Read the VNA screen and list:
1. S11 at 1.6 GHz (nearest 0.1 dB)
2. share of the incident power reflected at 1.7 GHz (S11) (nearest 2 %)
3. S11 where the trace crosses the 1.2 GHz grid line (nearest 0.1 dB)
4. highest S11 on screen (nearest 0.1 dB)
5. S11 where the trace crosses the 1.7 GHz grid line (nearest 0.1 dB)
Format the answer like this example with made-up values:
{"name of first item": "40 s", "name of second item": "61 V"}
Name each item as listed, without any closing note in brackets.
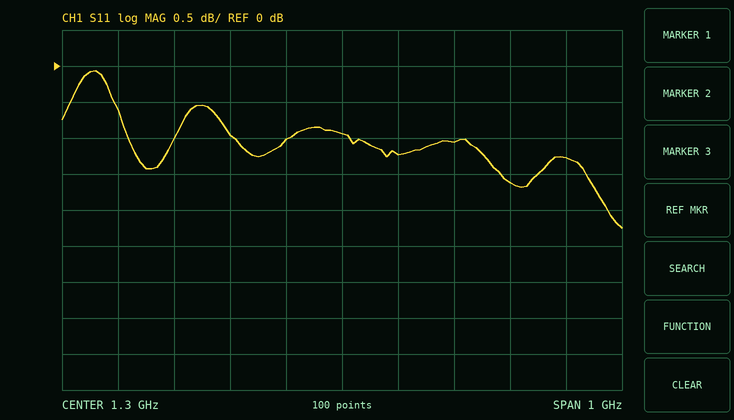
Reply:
{"S11 at 1.6 GHz": "-1.6 dB", "share of the incident power reflected at 1.7 GHz (S11)": "74 %", "S11 where the trace crosses the 1.2 GHz grid line": "-1.0 dB", "highest S11 on screen": "-0.1 dB", "S11 where the trace crosses the 1.7 GHz grid line": "-1.3 dB"}
